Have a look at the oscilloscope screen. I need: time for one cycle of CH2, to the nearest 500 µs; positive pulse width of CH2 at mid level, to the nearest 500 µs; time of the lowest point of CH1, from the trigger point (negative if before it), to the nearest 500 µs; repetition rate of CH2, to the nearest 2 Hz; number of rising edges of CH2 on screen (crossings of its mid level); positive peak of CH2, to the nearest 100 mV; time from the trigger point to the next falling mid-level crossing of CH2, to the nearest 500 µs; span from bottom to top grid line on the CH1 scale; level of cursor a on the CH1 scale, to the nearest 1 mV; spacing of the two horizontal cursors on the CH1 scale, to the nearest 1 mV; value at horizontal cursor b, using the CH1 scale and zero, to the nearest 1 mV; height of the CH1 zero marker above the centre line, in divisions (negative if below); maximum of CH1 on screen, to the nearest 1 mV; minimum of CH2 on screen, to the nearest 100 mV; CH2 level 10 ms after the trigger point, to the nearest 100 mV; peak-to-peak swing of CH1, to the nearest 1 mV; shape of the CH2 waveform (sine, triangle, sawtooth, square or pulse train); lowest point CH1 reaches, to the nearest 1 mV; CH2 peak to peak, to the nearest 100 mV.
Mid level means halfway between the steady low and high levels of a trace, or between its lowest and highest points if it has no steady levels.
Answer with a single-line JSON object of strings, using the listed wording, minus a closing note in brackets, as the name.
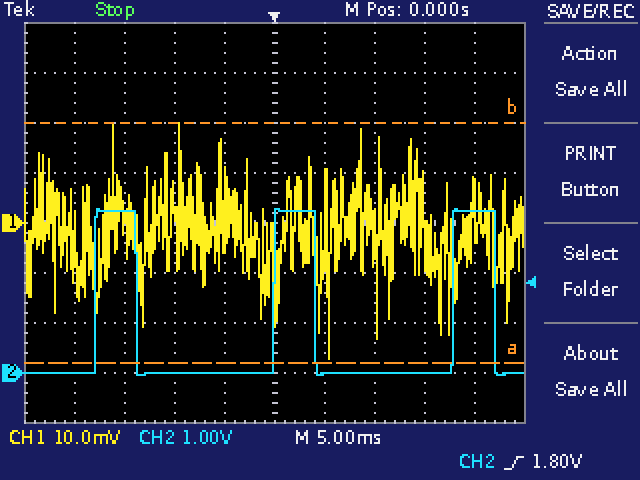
{"time for one cycle of CH2, to the nearest 500 µs": "18.0 ms", "positive pulse width of CH2 at mid level, to the nearest 500 µs": "4.0 ms", "time of the lowest point of CH1, from the trigger point (negative if before it), to the nearest 500 µs": "+5.5 ms", "repetition rate of CH2, to the nearest 2 Hz": "56 Hz", "number of rising edges of CH2 on screen": "3", "positive peak of CH2, to the nearest 100 mV": "3.3 V", "time from the trigger point to the next falling mid-level crossing of CH2, to the nearest 500 µs": "4.0 ms", "span from bottom to top grid line on the CH1 scale": "80 mV", "level of cursor a on the CH1 scale, to the nearest 1 mV": "-28 mV", "spacing of the two horizontal cursors on the CH1 scale, to the nearest 1 mV": "48 mV", "value at horizontal cursor b, using the CH1 scale and zero, to the nearest 1 mV": "20 mV", "height of the CH1 zero marker above the centre line, in divisions": "0.0 div", "maximum of CH1 on screen, to the nearest 1 mV": "20 mV", "minimum of CH2 on screen, to the nearest 100 mV": "0.0 V", "CH2 level 10 ms after the trigger point, to the nearest 100 mV": "0.0 V", "peak-to-peak swing of CH1, to the nearest 1 mV": "47 mV", "shape of the CH2 waveform": "pulse train", "lowest point CH1 reaches, to the nearest 1 mV": "-27 mV", "CH2 peak to peak, to the nearest 100 mV": "3.3 V"}
